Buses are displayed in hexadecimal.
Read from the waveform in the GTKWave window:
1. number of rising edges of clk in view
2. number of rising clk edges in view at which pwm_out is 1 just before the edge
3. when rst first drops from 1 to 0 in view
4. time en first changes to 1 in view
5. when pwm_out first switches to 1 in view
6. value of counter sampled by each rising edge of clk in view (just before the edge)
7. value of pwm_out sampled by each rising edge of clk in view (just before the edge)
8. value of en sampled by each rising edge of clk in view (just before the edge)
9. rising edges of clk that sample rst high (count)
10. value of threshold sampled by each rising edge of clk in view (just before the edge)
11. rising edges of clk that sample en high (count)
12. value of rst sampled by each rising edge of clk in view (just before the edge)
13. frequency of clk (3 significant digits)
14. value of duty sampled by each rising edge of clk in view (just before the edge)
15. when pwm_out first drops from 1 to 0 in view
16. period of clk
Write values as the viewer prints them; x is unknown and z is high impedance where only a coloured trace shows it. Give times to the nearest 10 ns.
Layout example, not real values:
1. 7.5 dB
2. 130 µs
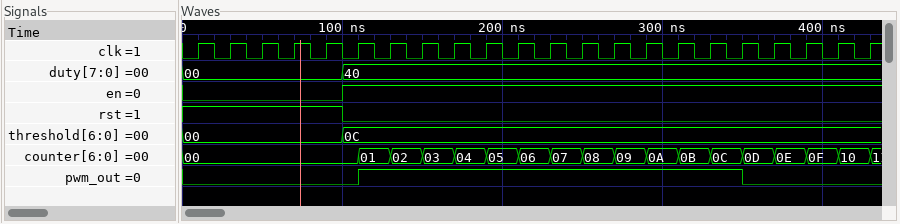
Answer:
1. 22
2. 12
3. 100 ns
4. 100 ns
5. 110 ns
6. 00, 00, 00, 00, 00, 00, 01, 02, 03, 04, 05, 06, 07, 08, 09, 0A, 0B, 0C, 0D, 0E, 0F, 10
7. 0 0 0 0 0 0 1 1 1 1 1 1 1 1 1 1 1 1 0 0 0 0
8. 0 0 0 0 0 1 1 1 1 1 1 1 1 1 1 1 1 1 1 1 1 1
9. 5
10. 00, 00, 00, 00, 00, 0C, 0C, 0C, 0C, 0C, 0C, 0C, 0C, 0C, 0C, 0C, 0C, 0C, 0C, 0C, 0C, 0C
11. 17
12. 1 1 1 1 1 0 0 0 0 0 0 0 0 0 0 0 0 0 0 0 0 0
13. 50.0 MHz
14. 00, 00, 00, 00, 00, 40, 40, 40, 40, 40, 40, 40, 40, 40, 40, 40, 40, 40, 40, 40, 40, 40
15. 350 ns
16. 20 ns
